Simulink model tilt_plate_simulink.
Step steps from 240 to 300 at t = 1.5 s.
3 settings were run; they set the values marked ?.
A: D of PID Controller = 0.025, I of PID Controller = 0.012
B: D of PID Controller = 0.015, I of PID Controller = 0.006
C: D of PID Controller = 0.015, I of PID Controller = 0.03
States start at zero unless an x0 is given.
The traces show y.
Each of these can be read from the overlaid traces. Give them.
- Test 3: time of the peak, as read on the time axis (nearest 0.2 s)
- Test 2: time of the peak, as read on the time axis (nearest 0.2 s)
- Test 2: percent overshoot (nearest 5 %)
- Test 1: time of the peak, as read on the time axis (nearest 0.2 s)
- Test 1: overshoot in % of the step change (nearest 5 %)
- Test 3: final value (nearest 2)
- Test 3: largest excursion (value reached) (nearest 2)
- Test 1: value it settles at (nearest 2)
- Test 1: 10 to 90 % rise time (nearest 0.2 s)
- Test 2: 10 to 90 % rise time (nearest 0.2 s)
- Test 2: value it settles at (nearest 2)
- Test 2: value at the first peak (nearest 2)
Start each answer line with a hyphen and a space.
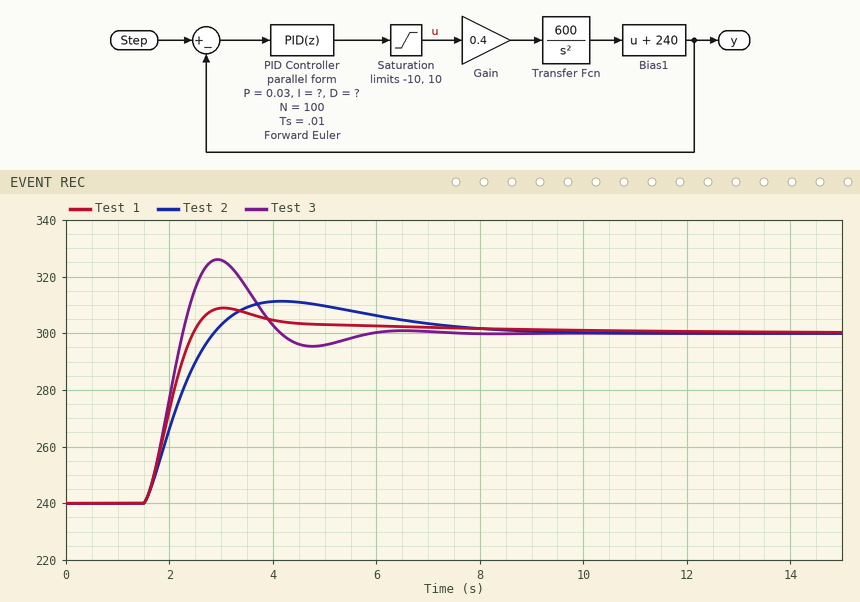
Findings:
- 3.0 s
- 4.2 s
- 20 %
- 3.0 s
- 15 %
- 300
- 326
- 300
- 0.6 s
- 1.0 s
- 300
- 312
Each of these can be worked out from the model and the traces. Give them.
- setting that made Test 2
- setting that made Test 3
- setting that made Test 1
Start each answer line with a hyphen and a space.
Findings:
- A
- C
- B
